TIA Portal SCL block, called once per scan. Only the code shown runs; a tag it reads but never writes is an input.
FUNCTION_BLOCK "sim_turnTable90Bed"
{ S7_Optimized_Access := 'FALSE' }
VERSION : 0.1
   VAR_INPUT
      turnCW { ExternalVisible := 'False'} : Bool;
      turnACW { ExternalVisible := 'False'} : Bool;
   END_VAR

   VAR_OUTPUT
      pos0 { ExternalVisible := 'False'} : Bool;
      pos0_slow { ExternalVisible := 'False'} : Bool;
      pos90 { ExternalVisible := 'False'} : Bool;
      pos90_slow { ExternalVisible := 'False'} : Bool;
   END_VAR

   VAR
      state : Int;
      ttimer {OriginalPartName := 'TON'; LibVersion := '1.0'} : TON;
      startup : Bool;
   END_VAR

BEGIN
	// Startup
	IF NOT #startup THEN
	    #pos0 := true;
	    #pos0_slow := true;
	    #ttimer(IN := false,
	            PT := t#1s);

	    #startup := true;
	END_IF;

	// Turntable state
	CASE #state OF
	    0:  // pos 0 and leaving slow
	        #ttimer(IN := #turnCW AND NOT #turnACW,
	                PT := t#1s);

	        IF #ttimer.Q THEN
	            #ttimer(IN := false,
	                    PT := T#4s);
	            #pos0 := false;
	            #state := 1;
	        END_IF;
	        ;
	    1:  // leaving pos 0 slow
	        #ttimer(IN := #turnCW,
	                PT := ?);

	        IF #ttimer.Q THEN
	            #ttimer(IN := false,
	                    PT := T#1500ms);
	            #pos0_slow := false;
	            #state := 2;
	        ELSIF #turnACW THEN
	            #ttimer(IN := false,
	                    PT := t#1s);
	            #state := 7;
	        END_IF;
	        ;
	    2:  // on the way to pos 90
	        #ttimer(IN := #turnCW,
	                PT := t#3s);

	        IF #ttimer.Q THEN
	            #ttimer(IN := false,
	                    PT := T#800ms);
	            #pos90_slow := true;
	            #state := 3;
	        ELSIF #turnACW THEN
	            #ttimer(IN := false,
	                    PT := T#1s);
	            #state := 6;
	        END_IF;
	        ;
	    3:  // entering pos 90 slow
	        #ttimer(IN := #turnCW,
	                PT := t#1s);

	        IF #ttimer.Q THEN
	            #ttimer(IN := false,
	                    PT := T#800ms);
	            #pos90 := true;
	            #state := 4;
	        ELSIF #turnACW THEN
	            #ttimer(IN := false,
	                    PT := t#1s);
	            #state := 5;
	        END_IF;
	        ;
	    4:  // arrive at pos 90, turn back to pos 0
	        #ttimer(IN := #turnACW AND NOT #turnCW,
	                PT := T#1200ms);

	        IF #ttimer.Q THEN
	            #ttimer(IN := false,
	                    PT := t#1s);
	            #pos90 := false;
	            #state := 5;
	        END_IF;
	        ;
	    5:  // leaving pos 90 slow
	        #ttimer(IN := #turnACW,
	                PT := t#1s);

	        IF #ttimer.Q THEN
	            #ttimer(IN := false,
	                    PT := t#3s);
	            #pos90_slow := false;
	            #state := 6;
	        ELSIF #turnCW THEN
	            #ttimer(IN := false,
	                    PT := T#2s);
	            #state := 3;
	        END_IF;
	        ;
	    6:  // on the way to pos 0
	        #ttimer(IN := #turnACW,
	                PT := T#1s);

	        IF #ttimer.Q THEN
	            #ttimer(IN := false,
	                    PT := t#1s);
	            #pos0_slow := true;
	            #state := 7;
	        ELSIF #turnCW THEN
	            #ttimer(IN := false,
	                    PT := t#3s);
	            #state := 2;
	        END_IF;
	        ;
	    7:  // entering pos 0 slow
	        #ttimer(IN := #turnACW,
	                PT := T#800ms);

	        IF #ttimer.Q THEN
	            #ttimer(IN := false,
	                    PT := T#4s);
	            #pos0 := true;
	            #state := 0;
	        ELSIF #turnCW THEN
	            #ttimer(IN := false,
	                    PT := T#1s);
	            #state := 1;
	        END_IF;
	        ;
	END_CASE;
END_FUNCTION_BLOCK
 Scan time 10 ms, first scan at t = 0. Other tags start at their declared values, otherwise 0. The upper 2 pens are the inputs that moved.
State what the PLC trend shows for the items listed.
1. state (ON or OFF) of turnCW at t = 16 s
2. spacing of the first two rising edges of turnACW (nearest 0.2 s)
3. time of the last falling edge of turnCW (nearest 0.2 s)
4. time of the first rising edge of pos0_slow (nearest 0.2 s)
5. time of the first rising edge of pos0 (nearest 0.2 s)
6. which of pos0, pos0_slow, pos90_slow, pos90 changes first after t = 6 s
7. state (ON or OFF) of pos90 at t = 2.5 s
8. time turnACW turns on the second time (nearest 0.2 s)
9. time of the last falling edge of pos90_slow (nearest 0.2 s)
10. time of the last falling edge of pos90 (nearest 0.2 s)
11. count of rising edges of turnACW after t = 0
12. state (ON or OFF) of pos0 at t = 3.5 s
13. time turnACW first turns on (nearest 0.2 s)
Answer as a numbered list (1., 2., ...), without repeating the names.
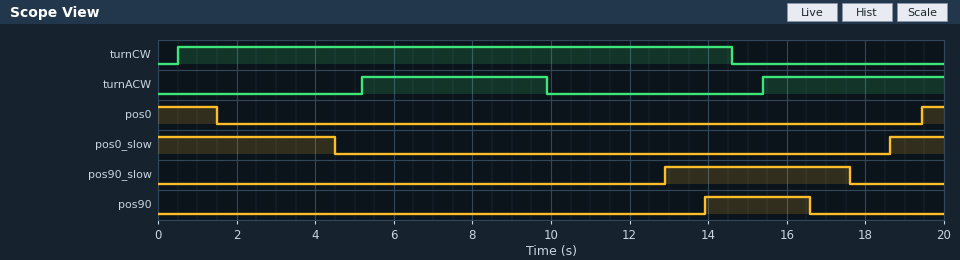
1. OFF
2. 10.2 s
3. 14.6 s
4. 18.6 s
5. 19.4 s
6. pos90_slow
7. OFF
8. 15.4 s
9. 17.6 s
10. 16.6 s
11. 2
12. OFF
13. 5.2 s
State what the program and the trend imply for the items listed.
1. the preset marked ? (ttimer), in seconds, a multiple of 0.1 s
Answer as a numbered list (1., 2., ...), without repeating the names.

1. 3.0 s
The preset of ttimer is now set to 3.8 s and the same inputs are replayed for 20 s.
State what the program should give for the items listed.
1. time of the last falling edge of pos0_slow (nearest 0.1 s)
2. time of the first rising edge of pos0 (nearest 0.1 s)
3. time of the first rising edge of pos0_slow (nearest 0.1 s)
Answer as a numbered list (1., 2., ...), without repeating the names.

1. 13.7 s
2. 17.2 s
3. 16.4 s
